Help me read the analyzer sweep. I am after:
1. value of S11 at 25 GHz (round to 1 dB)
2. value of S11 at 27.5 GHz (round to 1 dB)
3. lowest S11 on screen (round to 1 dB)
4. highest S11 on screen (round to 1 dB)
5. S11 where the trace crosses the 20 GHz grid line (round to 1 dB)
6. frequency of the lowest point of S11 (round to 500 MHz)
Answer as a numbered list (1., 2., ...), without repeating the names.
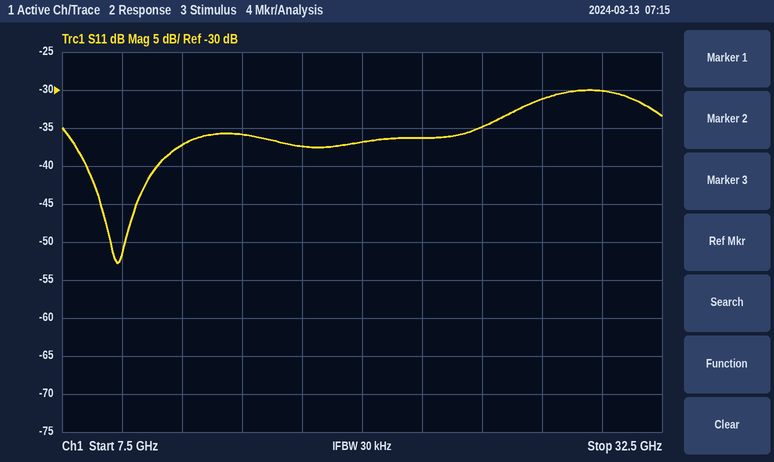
1. -35 dB
2. -31 dB
3. -53 dB
4. -30 dB
5. -37 dB
6. 10.0 GHz
